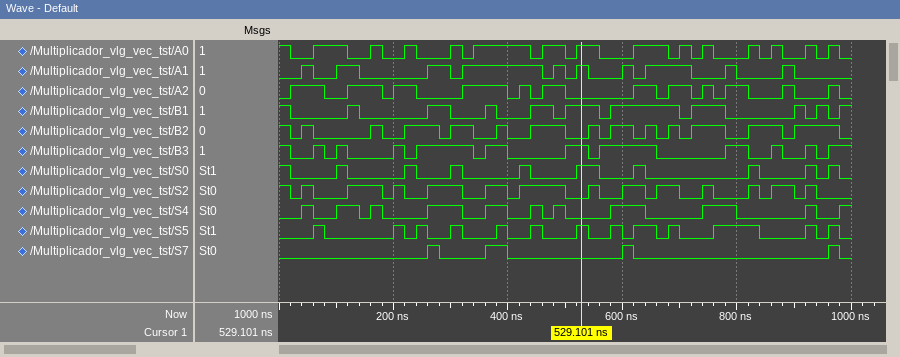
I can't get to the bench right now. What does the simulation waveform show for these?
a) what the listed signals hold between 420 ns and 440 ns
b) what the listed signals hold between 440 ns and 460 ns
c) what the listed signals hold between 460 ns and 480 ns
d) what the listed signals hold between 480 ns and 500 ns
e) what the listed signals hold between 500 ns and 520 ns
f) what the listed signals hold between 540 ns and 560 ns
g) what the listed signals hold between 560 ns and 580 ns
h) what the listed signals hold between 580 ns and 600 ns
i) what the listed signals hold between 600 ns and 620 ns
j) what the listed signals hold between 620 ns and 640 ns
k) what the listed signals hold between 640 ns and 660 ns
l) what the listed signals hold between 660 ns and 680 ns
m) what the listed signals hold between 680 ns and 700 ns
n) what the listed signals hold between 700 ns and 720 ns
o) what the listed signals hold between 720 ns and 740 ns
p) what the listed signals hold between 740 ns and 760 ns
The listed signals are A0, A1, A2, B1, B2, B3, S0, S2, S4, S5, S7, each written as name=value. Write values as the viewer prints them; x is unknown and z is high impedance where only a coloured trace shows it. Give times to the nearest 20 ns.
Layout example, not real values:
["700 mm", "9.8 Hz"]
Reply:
["A0=1, A1=1, A2=1, B1=0, B2=0, B3=0, S0=1, S2=1, S4=0, S5=0, S7=0", "A0=0, A1=1, A2=0, B1=1, B2=1, B3=0, S0=0, S2=1, S4=1, S5=1, S7=0", "A0=1, A1=0, A2=1, B1=1, B2=1, B3=0, S0=0, S2=1, S4=0, S5=0, S7=0", "A0=1, A1=1, A2=1, B1=0, B2=1, B3=0, S0=0, S2=1, S4=1, S5=0, S7=0", "A0=0, A1=0, A2=0, B1=1, B2=0, B3=1, S0=0, S2=0, S4=0, S5=0, S7=0", "A0=1, A1=0, A2=0, B1=1, B2=1, B3=0, S0=1, S2=1, S4=0, S5=0, S7=0", "A0=0, A1=0, A2=0, B1=0, B2=0, B3=1, S0=0, S2=0, S4=0, S5=0, S7=0", "A0=0, A1=0, A2=0, B1=1, B2=1, B3=1, S0=0, S2=0, S4=1, S5=1, S7=0", "A0=0, A1=1, A2=0, B1=1, B2=1, B3=1, S0=0, S2=1, S4=1, S5=0, S7=1", "A0=1, A1=0, A2=1, B1=1, B2=0, B3=1, S0=1, S2=1, S4=1, S5=1, S7=0", "A0=1, A1=1, A2=1, B1=1, B2=1, B3=1, S0=0, S2=0, S4=0, S5=1, S7=0", "A0=1, A1=1, A2=0, B1=1, B2=0, B3=0, S0=0, S2=1, S4=0, S5=0, S7=0", "A0=0, A1=1, A2=1, B1=1, B2=1, B3=0, S0=0, S2=1, S4=0, S5=1, S7=0", "A0=1, A1=1, A2=1, B1=0, B2=0, B3=0, S0=0, S2=0, S4=0, S5=0, S7=0", "A0=0, A1=0, A2=0, B1=1, B2=1, B3=0, S0=0, S2=0, S4=0, S5=0, S7=0", "A0=1, A1=0, A2=1, B1=1, B2=1, B3=0, S0=0, S2=1, S4=1, S5=0, S7=0"]
